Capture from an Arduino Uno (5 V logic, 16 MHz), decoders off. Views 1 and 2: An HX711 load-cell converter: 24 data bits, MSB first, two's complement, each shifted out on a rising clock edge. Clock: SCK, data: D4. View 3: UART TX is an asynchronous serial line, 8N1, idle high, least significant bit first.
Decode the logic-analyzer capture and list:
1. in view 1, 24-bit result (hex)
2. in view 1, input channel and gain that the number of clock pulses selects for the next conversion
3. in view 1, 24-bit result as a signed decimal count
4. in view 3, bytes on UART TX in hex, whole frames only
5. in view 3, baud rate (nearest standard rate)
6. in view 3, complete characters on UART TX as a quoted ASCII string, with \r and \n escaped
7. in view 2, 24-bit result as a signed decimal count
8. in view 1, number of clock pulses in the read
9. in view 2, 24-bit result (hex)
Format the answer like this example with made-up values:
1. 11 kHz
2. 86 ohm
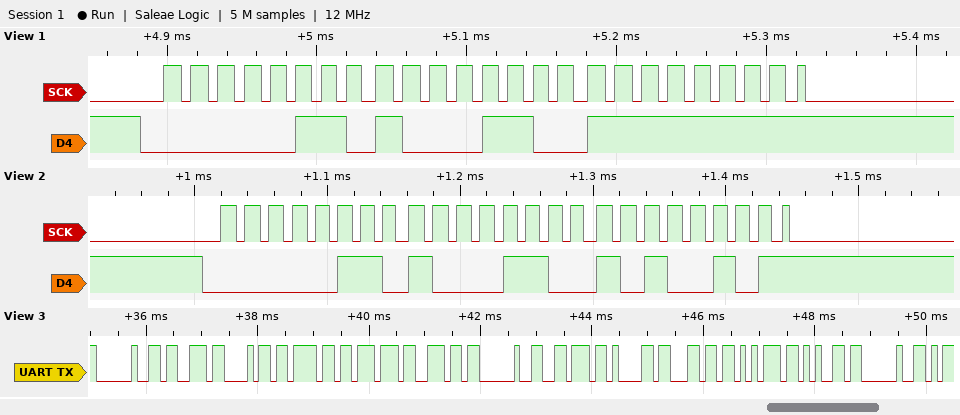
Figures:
1. 0x068CFF
2. channel A, gain 128
3. 429311
4. 20 73 68 6F 77 6E 20 76 61 6C 75 65 20
5. 9600 baud
6. " shown value "
7. 429221
8. 25
9. 0x068CA5
